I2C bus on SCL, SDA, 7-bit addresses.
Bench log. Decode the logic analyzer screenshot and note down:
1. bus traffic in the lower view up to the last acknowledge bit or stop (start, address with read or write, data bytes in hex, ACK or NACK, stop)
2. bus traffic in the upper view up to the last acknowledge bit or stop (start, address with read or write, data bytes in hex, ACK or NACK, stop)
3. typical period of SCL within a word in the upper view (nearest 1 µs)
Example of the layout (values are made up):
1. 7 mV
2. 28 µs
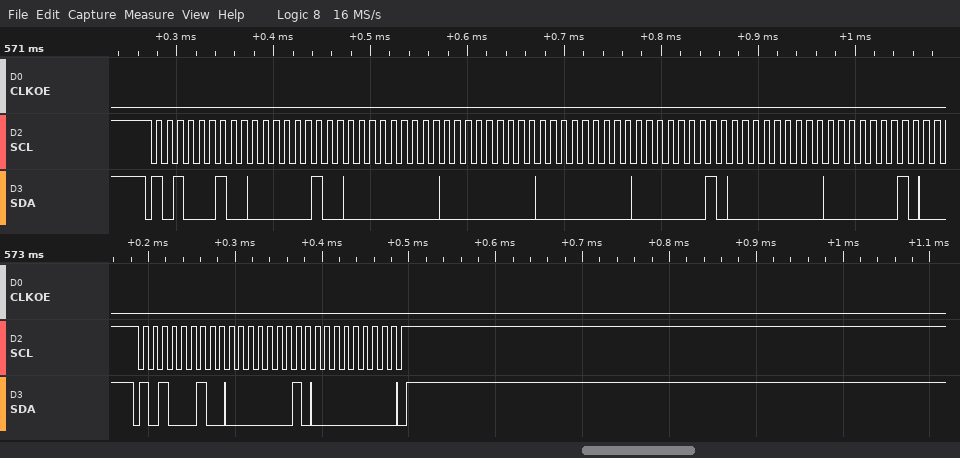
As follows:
1. start, address 51 write ACK, 01 ACK, 00 ACK, stop
2. start, address 51 write ACK, 02 ACK, 00 ACK, 00 ACK, 00 ACK, 01 ACK, 00 ACK, 01 ACK
3. 11 µs
